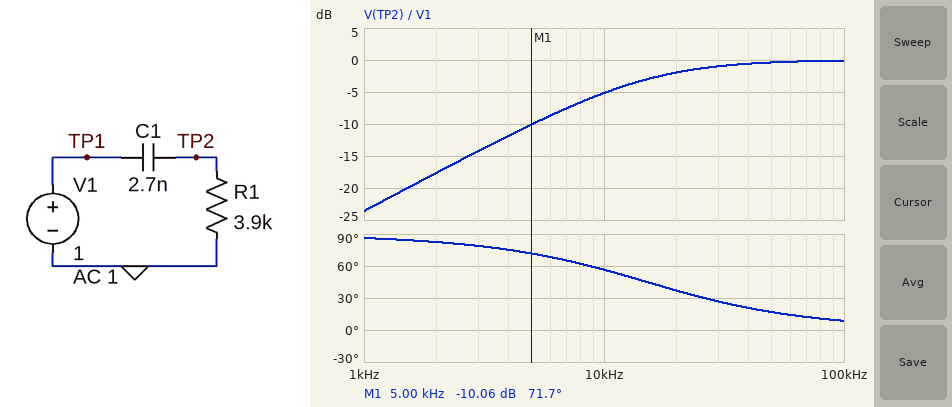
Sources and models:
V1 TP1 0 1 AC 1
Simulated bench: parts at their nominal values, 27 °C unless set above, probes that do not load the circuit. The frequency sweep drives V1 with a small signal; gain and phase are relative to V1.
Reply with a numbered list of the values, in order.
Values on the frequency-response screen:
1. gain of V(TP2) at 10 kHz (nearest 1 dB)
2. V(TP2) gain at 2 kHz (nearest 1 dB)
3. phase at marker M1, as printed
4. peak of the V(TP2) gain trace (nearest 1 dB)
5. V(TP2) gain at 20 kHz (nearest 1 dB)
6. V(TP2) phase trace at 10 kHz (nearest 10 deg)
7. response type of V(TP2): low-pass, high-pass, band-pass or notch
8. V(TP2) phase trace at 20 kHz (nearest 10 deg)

1. -5 dB
2. -18 dB
3. 71.7 deg
4. 0 dB
5. -2 dB
6. 60 deg
7. high-pass
8. 40 deg
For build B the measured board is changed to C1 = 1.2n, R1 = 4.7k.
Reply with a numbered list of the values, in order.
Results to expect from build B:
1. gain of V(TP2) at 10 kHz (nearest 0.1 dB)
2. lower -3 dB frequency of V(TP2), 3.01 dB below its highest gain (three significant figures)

1. -9.5 dB
2. 28.2 kHz
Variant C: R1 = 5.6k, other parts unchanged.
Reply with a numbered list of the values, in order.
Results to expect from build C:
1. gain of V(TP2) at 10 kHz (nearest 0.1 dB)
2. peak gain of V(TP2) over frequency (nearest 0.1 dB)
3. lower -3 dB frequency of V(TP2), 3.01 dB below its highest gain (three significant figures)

1. -3.2 dB
2. 0 dB
3. 10.5 kHz
